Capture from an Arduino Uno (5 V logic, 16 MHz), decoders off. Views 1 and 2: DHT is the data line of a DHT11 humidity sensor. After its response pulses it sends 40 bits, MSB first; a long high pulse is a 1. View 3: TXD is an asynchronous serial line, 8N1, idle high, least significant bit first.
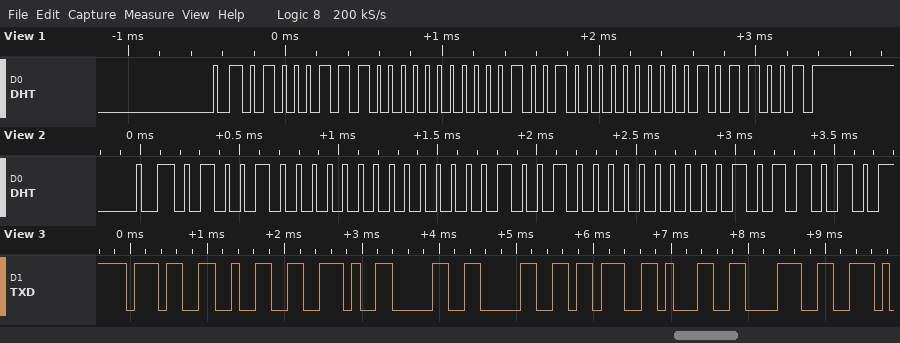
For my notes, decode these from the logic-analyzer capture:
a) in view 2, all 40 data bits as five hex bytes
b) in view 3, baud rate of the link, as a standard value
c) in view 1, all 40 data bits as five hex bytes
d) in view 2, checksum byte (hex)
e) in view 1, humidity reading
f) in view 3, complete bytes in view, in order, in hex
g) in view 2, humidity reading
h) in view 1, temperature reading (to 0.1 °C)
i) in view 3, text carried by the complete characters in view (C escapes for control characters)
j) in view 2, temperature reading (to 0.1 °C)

48 00 12 00 5A
9600 baud
47 00 12 00 59
0x5A
71 %
37 32 2E 30 30 3B 31 38
72 %
18.0 °C
"72.00;18"
18.0 °C
